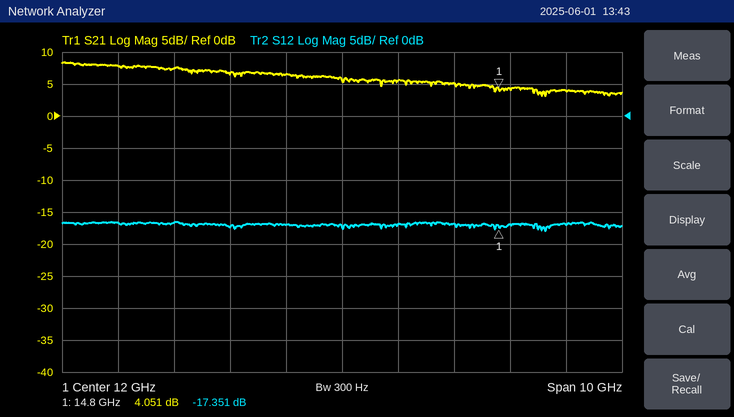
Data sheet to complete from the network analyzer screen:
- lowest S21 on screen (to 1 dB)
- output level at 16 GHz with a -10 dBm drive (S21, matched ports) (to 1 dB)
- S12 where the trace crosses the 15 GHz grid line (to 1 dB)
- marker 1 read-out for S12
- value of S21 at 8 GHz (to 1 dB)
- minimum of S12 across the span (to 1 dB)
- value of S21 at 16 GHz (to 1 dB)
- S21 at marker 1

3 dB
-6 dBm
-17 dB
-17.351 dB
8 dB
-18 dB
4 dB
4.051 dB
